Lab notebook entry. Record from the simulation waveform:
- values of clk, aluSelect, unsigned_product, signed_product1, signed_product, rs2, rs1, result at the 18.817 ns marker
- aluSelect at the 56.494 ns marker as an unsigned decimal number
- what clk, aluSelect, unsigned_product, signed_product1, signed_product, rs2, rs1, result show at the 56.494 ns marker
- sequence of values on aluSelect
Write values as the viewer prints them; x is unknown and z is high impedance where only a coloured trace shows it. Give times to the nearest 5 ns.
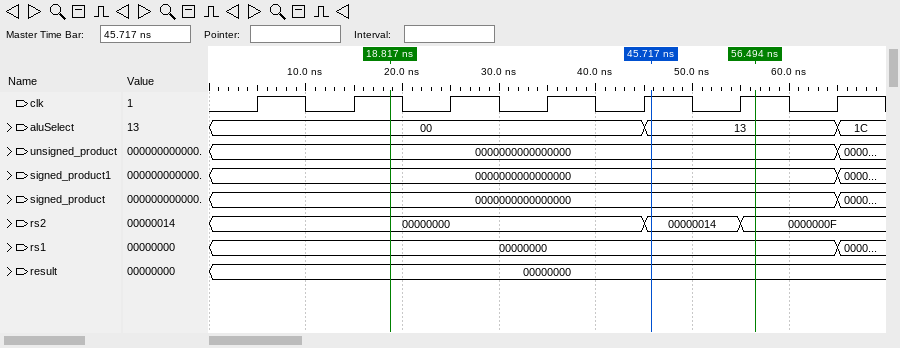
clk=1, aluSelect=00, unsigned_product=0000000000000000, signed_product1=0000000000000000, signed_product=0000000000000000, rs2=00000000, rs1=00000000, result=00000000
19
clk=1, aluSelect=13, unsigned_product=0000000000000000, signed_product1=0000000000000000, signed_product=0000000000000000, rs2=0000000F, rs1=00000000, result=00000000
00, 13, 1C
